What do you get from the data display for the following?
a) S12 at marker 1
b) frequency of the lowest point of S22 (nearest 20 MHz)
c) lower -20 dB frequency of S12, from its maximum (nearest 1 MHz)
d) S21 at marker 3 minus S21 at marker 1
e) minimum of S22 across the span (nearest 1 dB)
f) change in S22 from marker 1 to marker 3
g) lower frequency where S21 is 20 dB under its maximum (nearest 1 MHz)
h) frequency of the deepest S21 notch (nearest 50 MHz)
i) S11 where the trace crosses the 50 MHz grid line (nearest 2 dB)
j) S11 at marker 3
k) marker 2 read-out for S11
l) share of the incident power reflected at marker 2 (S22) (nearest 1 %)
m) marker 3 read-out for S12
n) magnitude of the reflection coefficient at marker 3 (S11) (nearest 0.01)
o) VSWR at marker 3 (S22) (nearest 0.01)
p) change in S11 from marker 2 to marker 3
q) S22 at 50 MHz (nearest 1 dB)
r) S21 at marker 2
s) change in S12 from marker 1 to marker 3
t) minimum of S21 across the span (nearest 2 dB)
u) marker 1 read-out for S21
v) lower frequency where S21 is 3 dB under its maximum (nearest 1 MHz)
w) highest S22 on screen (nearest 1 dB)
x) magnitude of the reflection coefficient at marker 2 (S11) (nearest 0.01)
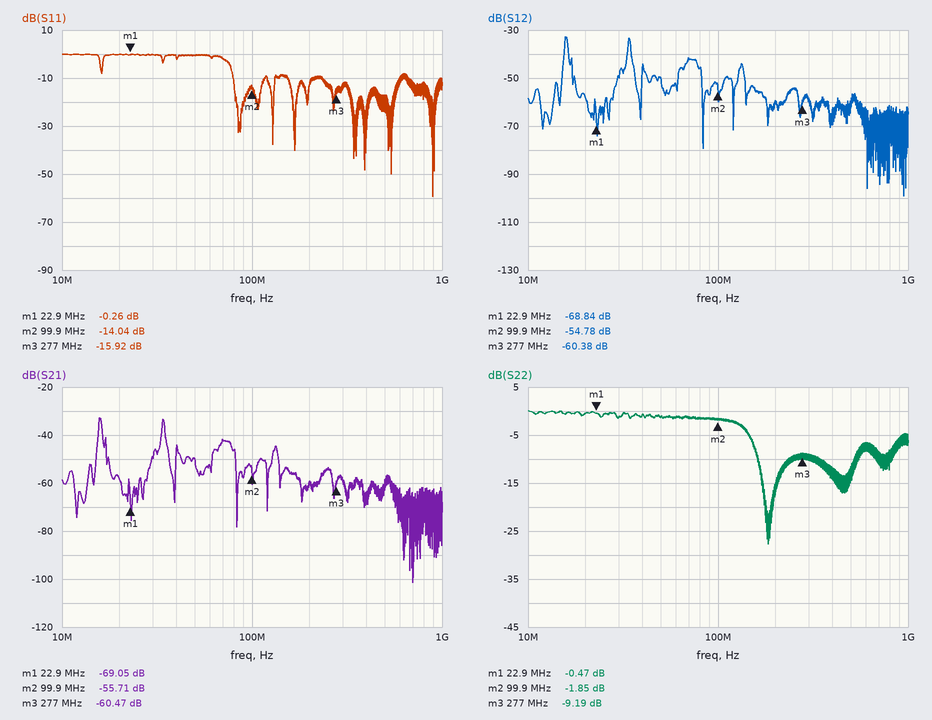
-68.84 dB
180 MHz
15 MHz
8.58 dB
-28 dB
-8.72 dB
15 MHz
700 MHz
0 dB
-15.92 dB
-14.04 dB
65 %
-60.38 dB
0.16
2.06
-1.88 dB
-1 dB
-55.71 dB
8.46 dB
-102 dB
-69.05 dB
16 MHz
0 dB
0.20
